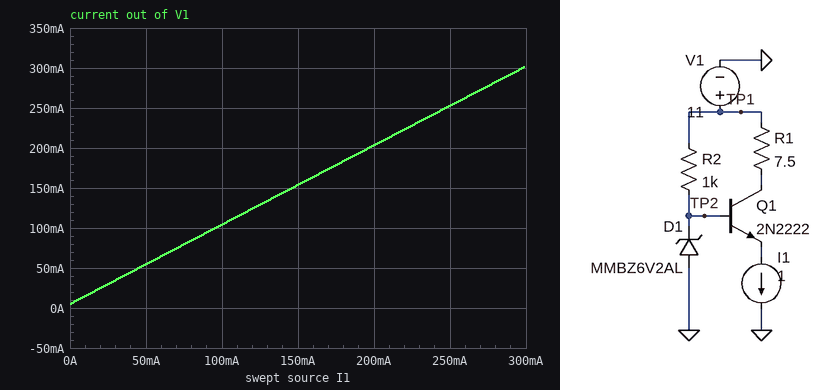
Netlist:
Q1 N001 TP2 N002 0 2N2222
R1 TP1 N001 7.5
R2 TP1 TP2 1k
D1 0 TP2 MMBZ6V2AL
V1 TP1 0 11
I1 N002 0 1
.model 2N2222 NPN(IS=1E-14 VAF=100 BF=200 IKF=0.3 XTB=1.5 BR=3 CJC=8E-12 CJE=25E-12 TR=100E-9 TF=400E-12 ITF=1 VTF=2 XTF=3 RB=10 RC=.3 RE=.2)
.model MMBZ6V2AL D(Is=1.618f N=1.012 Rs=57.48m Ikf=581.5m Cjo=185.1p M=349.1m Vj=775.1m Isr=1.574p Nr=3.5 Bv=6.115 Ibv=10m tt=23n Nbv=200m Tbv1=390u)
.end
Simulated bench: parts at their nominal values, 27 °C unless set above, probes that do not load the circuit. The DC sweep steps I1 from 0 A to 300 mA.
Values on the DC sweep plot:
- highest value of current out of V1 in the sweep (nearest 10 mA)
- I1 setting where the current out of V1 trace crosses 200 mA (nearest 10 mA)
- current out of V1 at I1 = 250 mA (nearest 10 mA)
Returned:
300 mA
200 mA
250 mA
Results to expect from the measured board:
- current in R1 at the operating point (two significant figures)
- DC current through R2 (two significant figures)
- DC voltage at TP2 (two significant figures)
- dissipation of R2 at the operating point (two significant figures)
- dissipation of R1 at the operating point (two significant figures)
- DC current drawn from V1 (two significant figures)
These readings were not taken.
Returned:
980 mA
12 mA
-770 mV
140 mW
7.2 W
990 mA
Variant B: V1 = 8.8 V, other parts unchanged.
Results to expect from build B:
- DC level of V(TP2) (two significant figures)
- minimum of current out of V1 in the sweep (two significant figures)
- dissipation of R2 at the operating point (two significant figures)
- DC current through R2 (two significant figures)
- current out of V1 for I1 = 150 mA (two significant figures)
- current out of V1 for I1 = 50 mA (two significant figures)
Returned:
-780 mV
2.7 mA
92 mW
9.6 mA
150 mA
52 mA
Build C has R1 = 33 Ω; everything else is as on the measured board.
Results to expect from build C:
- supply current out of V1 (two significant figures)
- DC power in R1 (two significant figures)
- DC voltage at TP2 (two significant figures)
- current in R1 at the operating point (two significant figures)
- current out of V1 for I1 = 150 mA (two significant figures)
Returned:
540 mA
9.1 W
-920 mV
530 mA
150 mA
